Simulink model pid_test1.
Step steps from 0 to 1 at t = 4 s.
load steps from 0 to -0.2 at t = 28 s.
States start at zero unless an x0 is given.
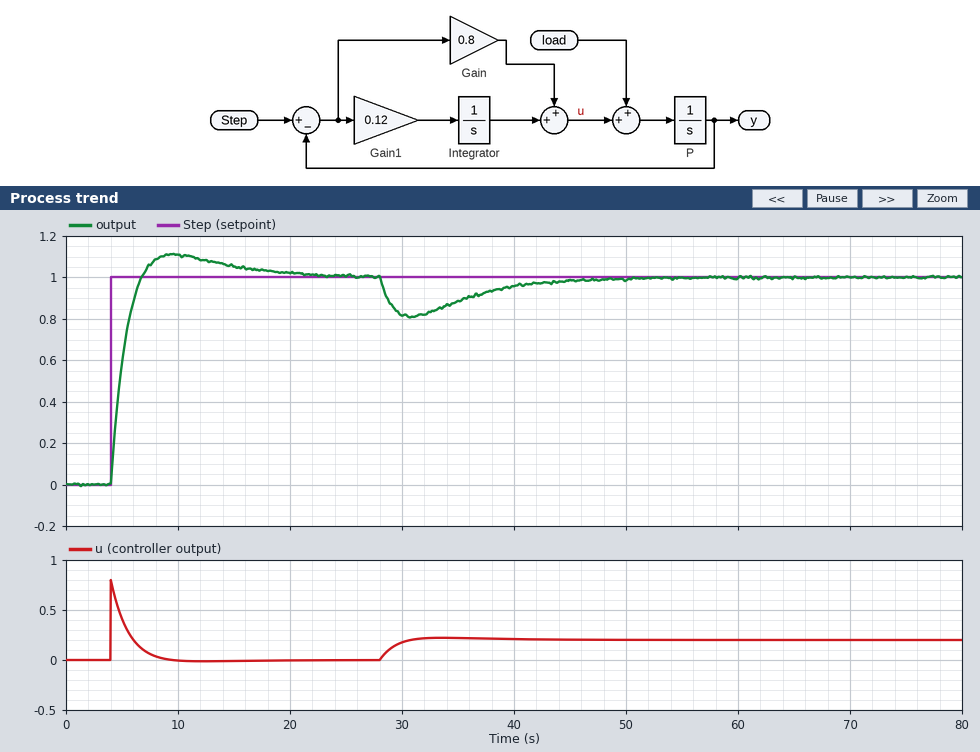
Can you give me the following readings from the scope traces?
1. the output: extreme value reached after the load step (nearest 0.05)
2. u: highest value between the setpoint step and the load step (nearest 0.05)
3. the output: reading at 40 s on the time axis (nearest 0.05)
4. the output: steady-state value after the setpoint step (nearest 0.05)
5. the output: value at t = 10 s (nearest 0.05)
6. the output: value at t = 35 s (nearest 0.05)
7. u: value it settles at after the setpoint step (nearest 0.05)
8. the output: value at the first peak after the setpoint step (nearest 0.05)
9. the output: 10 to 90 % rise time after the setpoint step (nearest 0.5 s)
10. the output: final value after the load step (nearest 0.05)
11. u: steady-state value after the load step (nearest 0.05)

0.80
0.80
0.95
1.00
1.10
0.90
0.00
1.10
2.0 s
1.00
0.20
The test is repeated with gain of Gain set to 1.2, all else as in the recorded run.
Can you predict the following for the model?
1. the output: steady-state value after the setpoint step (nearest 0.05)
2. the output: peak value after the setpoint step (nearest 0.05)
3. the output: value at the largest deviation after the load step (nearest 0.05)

1.00
1.05
0.85
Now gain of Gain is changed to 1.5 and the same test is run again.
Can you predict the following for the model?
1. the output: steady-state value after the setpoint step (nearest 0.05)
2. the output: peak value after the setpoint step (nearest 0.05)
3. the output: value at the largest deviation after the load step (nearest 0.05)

1.00
1.05
0.90
